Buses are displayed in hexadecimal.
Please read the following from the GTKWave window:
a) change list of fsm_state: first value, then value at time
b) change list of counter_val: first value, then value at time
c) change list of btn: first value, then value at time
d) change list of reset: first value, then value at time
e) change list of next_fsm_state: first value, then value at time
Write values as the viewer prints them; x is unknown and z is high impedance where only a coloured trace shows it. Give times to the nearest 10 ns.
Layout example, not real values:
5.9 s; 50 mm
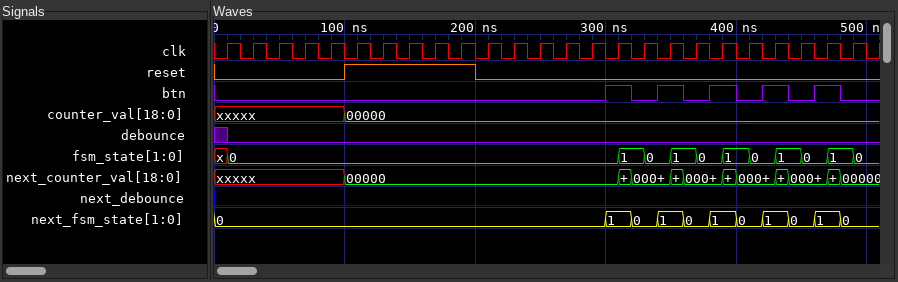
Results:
x, 0 at 10 ns, 1 at 310 ns, 0 at 330 ns, 1 at 350 ns, 0 at 370 ns, 1 at 390 ns, 0 at 410 ns, 1 at 430 ns, 0 at 450 ns, 1 at 470 ns, 0 at 490 ns; xxxxx, 00000 at 100 ns; 0, 1 at 300 ns, 0 at 320 ns, 1 at 340 ns, 0 at 360 ns, 1 at 380 ns, 0 at 400 ns, 1 at 420 ns, 0 at 440 ns, 1 at 460 ns, 0 at 480 ns; 0, 1 at 100 ns, 0 at 200 ns; 0, 1 at 300 ns, 0 at 320 ns, 1 at 340 ns, 0 at 360 ns, 1 at 380 ns, 0 at 400 ns, 1 at 420 ns, 0 at 440 ns, 1 at 460 ns, 0 at 480 ns
